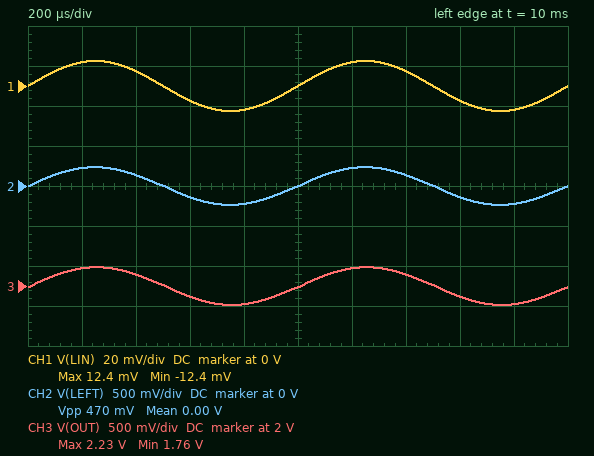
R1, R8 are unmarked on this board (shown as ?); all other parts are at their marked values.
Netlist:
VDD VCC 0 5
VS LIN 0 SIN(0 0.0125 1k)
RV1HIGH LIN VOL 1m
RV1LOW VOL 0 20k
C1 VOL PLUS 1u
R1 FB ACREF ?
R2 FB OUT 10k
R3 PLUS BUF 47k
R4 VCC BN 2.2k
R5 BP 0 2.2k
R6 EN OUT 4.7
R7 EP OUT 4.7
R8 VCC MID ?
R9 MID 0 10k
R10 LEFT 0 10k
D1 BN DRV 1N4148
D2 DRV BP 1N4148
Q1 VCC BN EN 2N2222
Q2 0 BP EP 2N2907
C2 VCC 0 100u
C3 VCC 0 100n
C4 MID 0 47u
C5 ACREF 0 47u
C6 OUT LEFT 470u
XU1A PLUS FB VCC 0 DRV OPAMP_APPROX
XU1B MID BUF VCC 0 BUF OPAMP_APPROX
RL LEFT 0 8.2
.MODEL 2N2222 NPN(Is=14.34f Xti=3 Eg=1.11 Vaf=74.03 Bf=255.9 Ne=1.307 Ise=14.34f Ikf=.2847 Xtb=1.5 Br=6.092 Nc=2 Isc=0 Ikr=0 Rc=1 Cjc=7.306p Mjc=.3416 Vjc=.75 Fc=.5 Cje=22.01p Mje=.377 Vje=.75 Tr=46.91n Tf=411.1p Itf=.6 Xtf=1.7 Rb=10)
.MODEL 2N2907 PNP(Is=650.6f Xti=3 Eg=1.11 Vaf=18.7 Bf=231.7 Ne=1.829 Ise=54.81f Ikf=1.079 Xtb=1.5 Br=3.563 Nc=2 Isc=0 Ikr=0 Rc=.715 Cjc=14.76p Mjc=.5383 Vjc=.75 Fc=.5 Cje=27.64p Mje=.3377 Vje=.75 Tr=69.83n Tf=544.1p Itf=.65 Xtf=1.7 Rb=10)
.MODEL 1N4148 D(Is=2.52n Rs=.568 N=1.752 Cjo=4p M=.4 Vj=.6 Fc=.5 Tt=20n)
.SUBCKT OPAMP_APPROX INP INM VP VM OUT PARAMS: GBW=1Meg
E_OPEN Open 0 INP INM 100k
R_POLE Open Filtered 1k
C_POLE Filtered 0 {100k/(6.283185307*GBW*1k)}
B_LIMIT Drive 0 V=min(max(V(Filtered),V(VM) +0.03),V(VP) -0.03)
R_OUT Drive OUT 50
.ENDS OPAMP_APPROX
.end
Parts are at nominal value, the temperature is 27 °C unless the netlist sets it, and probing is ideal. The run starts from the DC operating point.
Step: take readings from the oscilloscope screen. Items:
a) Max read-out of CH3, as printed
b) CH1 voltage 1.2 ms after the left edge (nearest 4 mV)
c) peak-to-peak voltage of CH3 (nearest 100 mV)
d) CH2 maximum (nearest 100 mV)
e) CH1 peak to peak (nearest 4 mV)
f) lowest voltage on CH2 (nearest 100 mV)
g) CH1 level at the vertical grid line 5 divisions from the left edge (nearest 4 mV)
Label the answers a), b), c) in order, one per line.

a) 2.23 V
b) 12 mV
c) 500 mV
d) 200 mV
e) 24 mV
f) -200 mV
g) 0 V
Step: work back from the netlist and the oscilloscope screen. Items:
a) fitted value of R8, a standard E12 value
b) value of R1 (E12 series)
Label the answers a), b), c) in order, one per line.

a) 15 kΩ
b) 560 Ω
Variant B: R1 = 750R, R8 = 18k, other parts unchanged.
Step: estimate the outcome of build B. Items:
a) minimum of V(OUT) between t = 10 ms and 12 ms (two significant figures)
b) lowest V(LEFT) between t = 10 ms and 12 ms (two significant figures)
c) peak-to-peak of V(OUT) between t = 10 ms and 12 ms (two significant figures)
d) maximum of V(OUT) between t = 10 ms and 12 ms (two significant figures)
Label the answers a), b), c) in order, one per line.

a) 1.6 V
b) -180 mV
c) 360 mV
d) 2.0 V
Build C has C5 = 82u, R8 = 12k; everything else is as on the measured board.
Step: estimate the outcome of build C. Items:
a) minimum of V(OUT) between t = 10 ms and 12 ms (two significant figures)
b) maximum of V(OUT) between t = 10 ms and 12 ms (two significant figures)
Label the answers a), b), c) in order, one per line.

a) 2.0 V
b) 2.5 V
